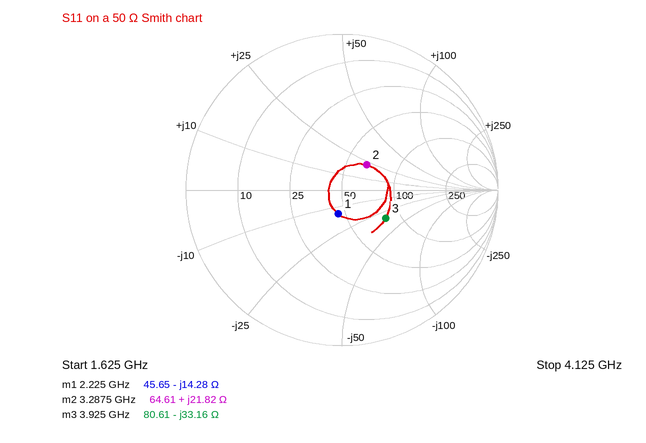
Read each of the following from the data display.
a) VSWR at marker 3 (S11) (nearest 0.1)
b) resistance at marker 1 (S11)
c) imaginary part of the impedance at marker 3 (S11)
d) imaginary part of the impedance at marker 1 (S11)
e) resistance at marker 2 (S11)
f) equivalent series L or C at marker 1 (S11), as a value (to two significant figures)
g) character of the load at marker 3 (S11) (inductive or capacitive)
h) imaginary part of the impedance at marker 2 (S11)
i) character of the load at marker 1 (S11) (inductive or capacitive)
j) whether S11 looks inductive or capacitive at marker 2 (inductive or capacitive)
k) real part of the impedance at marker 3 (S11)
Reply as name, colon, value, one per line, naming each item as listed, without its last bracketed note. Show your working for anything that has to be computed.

VSWR at marker 3 (S11): 2.0
resistance at marker 1: 45.65 Ω
imaginary part of the impedance at marker 3: -33.16 Ω
imaginary part of the impedance at marker 1: -14.28 Ω
resistance at marker 2: 64.61 Ω
equivalent series L or C at marker 1 (S11), as a value: C = 1/(2π × 2.225 GHz × 14.28 Ω) ≈ 5.0 pF
character of the load at marker 3 (S11): capacitive
imaginary part of the impedance at marker 2: +21.82 Ω
character of the load at marker 1 (S11): capacitive
whether S11 looks inductive or capacitive at marker 2: inductive
real part of the impedance at marker 3: 80.61 Ω
